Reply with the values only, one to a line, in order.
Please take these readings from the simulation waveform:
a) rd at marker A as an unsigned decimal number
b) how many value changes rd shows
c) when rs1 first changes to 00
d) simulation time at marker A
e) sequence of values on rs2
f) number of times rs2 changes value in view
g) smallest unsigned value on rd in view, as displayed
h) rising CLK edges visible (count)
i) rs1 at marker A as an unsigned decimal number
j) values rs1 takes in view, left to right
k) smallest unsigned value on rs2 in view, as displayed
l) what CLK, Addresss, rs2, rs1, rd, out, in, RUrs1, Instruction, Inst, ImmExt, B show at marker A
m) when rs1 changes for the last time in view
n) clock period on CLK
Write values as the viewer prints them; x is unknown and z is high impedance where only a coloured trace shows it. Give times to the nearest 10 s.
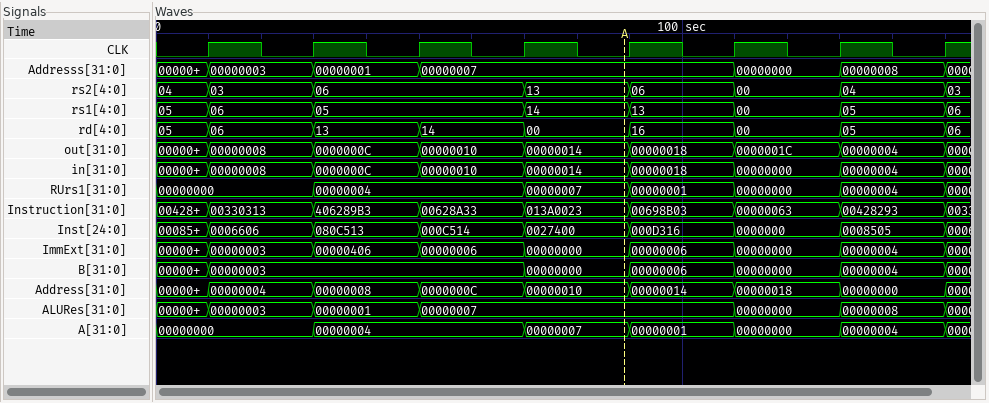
0
8
110 s
90 s
04, 03, 06, 13, 06, 00, 04, 03
7
00
8
20
05, 06, 05, 14, 13, 00, 05, 06
00
CLK=0, Addresss=00000007, rs2=13, rs1=14, rd=00, out=00000014, in=00000014, RUrs1=00000007, Instruction=013A0023, Inst=0027400, ImmExt=00000000, B=00000000
150 s
20 s
